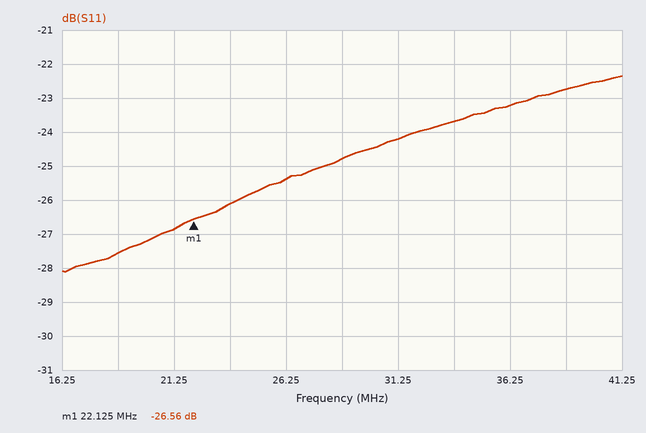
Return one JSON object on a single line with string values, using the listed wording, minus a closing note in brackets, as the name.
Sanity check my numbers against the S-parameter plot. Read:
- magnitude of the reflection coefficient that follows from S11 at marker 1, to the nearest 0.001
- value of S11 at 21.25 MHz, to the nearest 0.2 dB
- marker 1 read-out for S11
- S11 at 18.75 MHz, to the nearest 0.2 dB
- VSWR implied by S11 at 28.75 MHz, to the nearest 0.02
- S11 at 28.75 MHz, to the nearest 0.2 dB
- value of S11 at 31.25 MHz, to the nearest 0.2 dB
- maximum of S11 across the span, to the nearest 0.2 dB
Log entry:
{"magnitude of the reflection coefficient that follows from S11 at marker 1, to the nearest 0.001": "0.047", "value of S11 at 21.25 MHz, to the nearest 0.2 dB": "-26.8 dB", "marker 1 read-out for S11": "-26.56 dB", "S11 at 18.75 MHz, to the nearest 0.2 dB": "-27.6 dB", "VSWR implied by S11 at 28.75 MHz, to the nearest 0.02": "1.12", "S11 at 28.75 MHz, to the nearest 0.2 dB": "-24.8 dB", "value of S11 at 31.25 MHz, to the nearest 0.2 dB": "-24.2 dB", "maximum of S11 across the span, to the nearest 0.2 dB": "-22.4 dB"}
